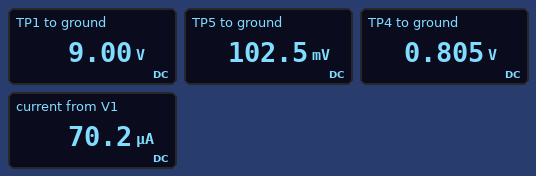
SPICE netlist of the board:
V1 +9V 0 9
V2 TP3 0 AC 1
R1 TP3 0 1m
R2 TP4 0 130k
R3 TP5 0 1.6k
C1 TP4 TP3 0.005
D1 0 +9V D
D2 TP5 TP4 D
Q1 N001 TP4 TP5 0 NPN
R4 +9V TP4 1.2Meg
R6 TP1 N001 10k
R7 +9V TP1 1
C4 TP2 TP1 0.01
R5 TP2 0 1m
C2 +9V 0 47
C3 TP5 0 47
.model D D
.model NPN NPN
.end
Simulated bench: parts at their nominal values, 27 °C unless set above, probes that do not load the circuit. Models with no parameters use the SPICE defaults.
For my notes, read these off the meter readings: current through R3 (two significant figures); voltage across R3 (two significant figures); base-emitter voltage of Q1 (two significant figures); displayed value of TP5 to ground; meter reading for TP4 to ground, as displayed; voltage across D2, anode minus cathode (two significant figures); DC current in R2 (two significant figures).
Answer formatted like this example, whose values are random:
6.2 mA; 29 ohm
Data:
64 µA; 100 mV; 700 mV; 102.5 mV; 0.805 V; -700 mV; 6.2 µA
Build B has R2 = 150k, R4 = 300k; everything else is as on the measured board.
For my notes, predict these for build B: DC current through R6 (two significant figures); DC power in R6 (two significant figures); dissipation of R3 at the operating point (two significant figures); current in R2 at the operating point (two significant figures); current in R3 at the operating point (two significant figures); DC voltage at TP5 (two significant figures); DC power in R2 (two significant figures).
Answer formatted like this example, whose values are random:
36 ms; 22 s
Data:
760 µA; 5.8 mW; 950 µW; 13 µA; 770 µA; 1.2 V; 27 µW
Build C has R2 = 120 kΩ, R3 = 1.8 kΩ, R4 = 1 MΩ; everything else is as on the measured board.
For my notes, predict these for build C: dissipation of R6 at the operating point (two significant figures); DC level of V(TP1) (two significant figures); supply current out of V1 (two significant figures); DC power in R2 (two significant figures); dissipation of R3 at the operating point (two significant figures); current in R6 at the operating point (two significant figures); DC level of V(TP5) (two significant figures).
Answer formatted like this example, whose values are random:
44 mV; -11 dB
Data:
77 µW; 9.0 V; 96 µA; 6.3 µW; 14 µW; 88 µA; 160 mV
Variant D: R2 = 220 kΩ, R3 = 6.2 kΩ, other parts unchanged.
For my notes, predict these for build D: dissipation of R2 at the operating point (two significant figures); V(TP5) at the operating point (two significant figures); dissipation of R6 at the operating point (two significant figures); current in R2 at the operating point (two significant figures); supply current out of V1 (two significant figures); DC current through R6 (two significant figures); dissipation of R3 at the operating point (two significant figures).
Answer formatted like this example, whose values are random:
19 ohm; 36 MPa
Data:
7.0 µW; 530 mV; 71 µW; 5.6 µA; 91 µA; 84 µA; 45 µW
